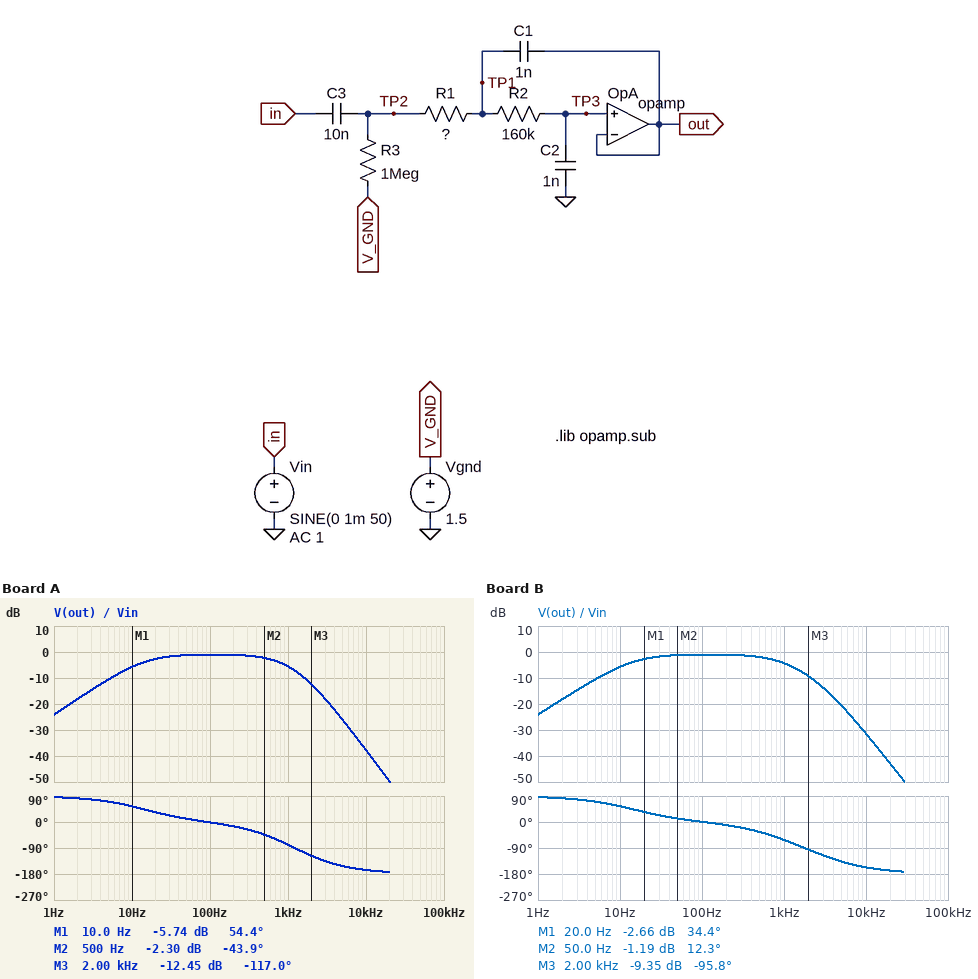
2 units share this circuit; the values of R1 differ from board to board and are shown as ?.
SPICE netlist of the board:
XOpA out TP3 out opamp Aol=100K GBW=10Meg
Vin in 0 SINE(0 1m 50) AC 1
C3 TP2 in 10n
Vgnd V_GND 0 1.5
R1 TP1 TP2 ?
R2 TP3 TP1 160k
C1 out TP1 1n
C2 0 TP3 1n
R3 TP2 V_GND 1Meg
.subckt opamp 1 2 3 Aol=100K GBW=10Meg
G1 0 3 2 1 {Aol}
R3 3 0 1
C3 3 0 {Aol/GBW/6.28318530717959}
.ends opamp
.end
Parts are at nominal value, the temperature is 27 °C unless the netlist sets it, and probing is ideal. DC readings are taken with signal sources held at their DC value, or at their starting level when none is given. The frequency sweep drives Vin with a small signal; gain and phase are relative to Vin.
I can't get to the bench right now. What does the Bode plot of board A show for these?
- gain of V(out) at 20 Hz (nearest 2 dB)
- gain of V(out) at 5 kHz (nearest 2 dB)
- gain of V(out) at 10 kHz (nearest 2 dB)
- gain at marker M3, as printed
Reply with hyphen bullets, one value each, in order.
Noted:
- -2 dB
- -26 dB
- -38 dB
- -12.45 dB
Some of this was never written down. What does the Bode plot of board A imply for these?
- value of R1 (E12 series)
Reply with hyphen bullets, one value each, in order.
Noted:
- 120 kΩ
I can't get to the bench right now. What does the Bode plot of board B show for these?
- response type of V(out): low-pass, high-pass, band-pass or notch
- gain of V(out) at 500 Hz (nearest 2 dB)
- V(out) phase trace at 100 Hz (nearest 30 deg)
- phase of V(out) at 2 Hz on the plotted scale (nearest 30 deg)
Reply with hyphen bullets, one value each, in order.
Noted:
- band-pass
- -2 dB
- 0 deg
- 90 deg
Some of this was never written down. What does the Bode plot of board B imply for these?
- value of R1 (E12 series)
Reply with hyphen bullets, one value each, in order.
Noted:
- 56 kΩ
